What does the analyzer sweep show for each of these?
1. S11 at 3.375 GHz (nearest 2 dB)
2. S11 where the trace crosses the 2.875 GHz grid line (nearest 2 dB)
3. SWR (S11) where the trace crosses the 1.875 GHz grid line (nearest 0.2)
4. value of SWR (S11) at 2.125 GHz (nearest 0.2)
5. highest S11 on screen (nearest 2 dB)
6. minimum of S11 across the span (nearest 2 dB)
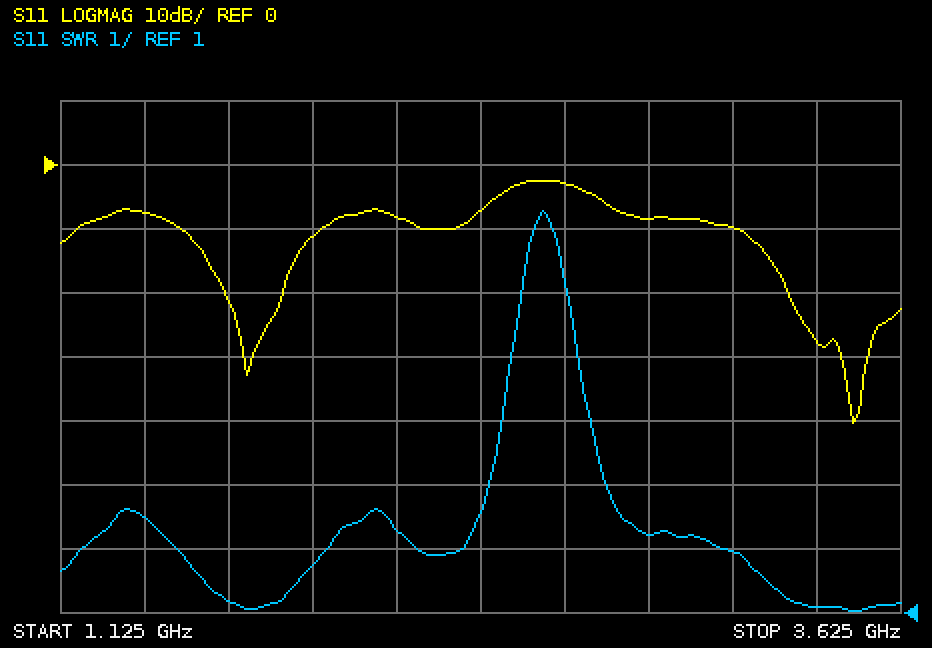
-28 dB
-8 dB
1.8
2.2
-2 dB
-40 dB
